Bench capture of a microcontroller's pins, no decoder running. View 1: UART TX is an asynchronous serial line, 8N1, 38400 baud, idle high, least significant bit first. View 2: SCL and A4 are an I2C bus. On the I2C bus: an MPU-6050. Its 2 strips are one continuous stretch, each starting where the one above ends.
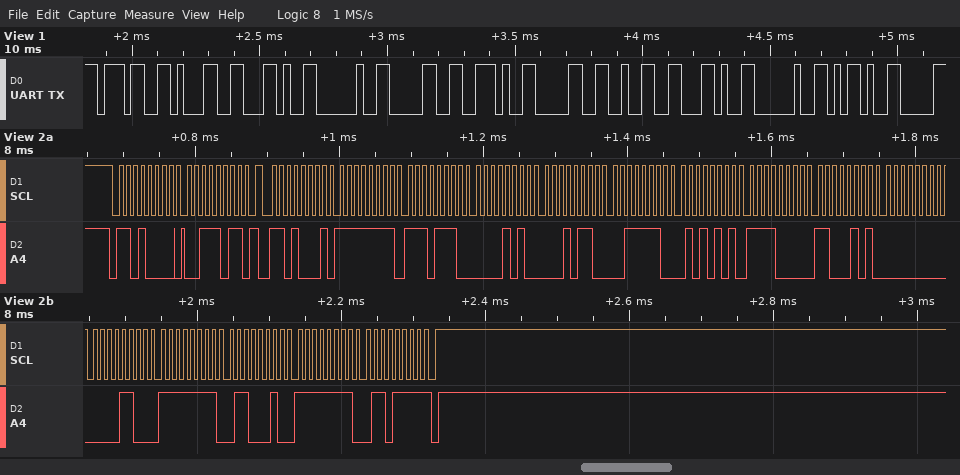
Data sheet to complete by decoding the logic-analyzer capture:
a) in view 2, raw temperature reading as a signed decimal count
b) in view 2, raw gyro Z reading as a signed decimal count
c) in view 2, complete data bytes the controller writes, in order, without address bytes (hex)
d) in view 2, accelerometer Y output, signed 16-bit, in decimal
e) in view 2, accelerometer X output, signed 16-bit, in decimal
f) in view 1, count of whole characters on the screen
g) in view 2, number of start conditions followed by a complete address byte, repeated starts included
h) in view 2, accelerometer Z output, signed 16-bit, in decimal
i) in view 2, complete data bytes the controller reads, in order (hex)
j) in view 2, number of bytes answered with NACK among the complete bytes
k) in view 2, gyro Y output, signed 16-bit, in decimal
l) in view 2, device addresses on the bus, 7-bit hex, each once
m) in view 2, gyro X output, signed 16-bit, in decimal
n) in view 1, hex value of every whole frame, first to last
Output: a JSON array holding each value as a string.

["-3899", "-145", "3B", "2582", "-18", "11", "2", "15957", "FF EE 0A 16 3E 55 F0 C5 00 0C FF 62 FF 6F", "1", "-158", "0x68", "12", "37 31 2C 20 30 2E 30 32 2C 20 2D"]
